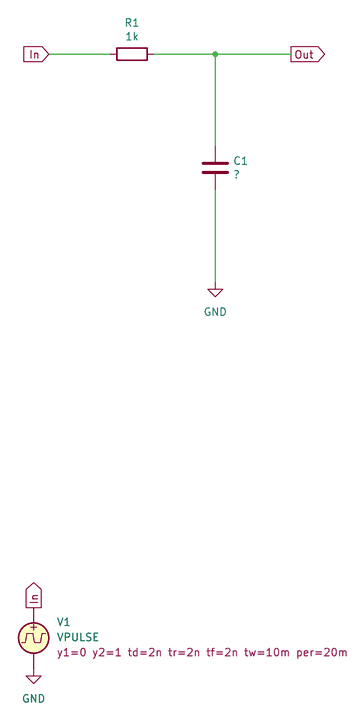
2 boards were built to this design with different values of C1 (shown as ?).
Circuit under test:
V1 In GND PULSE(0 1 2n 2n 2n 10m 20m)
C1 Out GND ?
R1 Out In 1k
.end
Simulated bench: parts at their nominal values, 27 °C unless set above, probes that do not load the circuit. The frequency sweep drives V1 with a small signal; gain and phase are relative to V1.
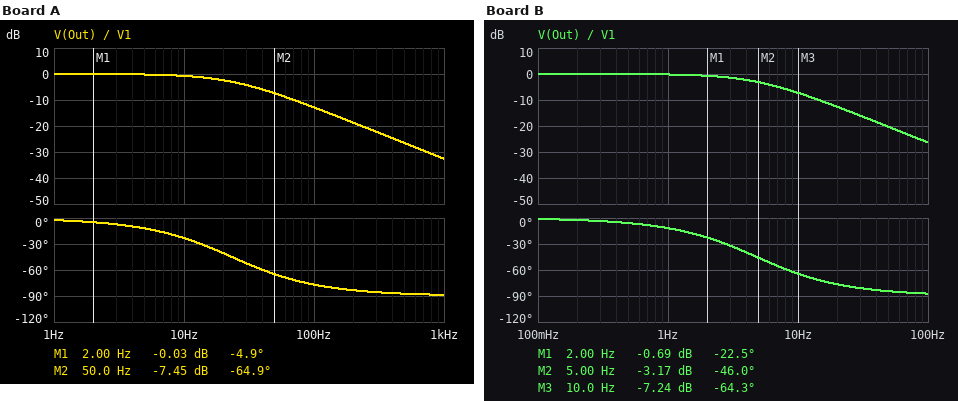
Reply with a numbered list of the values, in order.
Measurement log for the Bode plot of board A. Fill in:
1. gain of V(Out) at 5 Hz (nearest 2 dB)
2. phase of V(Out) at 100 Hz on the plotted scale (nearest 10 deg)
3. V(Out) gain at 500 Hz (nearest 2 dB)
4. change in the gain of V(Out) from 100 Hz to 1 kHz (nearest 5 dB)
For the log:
1. 0 dB
2. -80 deg
3. -26 dB
4. -20 dB
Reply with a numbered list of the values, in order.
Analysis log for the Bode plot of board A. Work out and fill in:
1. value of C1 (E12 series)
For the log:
1. 6.8 µF
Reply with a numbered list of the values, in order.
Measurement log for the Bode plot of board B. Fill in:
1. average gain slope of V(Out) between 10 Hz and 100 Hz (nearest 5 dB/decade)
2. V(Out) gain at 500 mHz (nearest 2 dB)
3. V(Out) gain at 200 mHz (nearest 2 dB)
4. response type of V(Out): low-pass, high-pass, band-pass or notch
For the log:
1. -20 dB/decade
2. 0 dB
3. 0 dB
4. low-pass
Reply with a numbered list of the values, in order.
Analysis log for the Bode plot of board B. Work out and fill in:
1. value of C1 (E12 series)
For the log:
1. 33 µF
